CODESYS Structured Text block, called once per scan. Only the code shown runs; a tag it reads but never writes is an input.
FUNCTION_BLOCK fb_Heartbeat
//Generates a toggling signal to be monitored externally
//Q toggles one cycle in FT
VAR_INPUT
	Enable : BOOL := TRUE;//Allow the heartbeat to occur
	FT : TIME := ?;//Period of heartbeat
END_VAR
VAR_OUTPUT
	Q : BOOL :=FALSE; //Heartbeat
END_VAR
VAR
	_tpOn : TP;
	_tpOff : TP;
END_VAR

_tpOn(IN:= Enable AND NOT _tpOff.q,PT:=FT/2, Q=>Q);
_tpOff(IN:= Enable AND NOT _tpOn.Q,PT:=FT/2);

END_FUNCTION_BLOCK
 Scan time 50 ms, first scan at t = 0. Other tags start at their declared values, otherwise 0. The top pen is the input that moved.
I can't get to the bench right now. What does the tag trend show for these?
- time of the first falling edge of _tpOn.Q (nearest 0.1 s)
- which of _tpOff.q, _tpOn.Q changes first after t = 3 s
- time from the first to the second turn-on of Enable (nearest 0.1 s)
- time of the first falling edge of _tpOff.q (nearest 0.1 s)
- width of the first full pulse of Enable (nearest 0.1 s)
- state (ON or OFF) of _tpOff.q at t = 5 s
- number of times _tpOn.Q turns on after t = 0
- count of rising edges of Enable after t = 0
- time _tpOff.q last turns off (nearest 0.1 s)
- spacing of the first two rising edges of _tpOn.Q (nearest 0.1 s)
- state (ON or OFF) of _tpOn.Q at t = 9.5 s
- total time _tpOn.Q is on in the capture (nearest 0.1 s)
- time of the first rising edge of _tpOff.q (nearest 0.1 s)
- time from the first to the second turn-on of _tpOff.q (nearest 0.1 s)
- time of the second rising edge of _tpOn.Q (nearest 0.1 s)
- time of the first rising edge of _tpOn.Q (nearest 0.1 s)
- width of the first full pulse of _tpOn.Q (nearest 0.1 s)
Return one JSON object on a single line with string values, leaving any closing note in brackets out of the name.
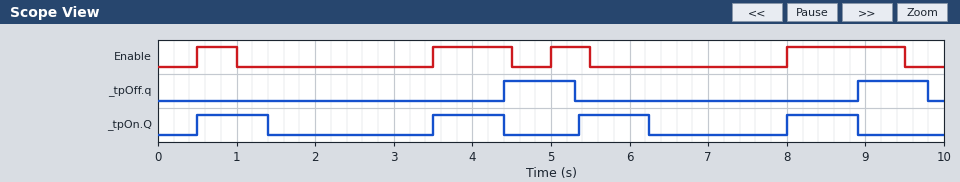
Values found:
{"time of the first falling edge of _tpOn.Q": "1.4 s", "which of _tpOff.q, _tpOn.Q changes first after t = 3 s": "_tpOn.Q", "time from the first to the second turn-on of Enable": "3.0 s", "time of the first falling edge of _tpOff.q": "5.3 s", "width of the first full pulse of Enable": "0.5 s", "state (ON or OFF) of _tpOff.q at t = 5 s": "ON", "number of times _tpOn.Q turns on after t = 0": "4", "count of rising edges of Enable after t = 0": "4", "time _tpOff.q last turns off": "9.8 s", "spacing of the first two rising edges of _tpOn.Q": "3.0 s", "state (ON or OFF) of _tpOn.Q at t = 9.5 s": "OFF", "total time _tpOn.Q is on in the capture": "3.6 s", "time of the first rising edge of _tpOff.q": "4.4 s", "time from the first to the second turn-on of _tpOff.q": "4.5 s", "time of the second rising edge of _tpOn.Q": "3.5 s", "time of the first rising edge of _tpOn.Q": "0.5 s", "width of the first full pulse of _tpOn.Q": "0.9 s"}
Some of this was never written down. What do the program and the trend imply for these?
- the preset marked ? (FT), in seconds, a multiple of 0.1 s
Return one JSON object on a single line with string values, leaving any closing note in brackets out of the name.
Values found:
{"the preset marked ? (FT), in seconds, a multiple of 0.1 s": "1.8 s"}
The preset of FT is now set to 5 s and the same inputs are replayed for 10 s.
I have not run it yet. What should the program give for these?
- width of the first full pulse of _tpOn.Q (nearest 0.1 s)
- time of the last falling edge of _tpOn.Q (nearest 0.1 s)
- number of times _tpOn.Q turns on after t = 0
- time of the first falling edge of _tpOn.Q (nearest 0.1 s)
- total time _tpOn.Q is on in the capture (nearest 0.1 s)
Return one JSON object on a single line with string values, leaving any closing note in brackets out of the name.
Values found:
{"width of the first full pulse of _tpOn.Q": "2.5 s", "time of the last falling edge of _tpOn.Q": "6.0 s", "number of times _tpOn.Q turns on after t = 0": "3", "time of the first falling edge of _tpOn.Q": "3.0 s", "total time _tpOn.Q is on in the capture": "7.0 s"}
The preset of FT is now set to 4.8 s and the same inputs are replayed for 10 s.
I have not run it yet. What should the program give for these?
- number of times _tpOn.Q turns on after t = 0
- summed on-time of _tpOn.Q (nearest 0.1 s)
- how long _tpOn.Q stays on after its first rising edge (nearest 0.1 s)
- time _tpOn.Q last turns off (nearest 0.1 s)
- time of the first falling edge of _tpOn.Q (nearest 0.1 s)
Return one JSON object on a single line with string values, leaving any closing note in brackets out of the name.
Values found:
{"number of times _tpOn.Q turns on after t = 0": "3", "summed on-time of _tpOn.Q": "6.8 s", "how long _tpOn.Q stays on after its first rising edge": "2.4 s", "time _tpOn.Q last turns off": "5.9 s", "time of the first falling edge of _tpOn.Q": "2.9 s"}
